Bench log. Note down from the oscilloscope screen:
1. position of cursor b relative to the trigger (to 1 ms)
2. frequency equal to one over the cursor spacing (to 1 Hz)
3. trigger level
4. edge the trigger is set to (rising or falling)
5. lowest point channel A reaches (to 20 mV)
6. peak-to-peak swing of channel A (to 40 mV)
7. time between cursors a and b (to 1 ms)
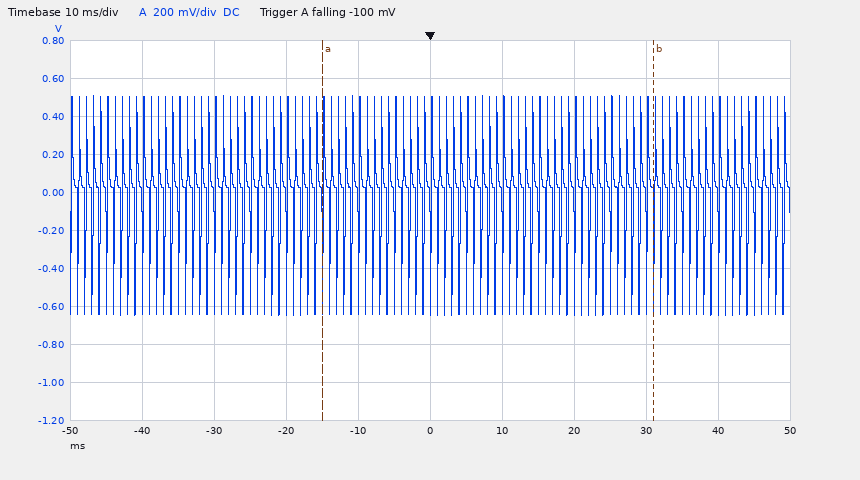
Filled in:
+31 ms
22 Hz
-100 mV
falling
-640 mV
1.16 V
46 ms
